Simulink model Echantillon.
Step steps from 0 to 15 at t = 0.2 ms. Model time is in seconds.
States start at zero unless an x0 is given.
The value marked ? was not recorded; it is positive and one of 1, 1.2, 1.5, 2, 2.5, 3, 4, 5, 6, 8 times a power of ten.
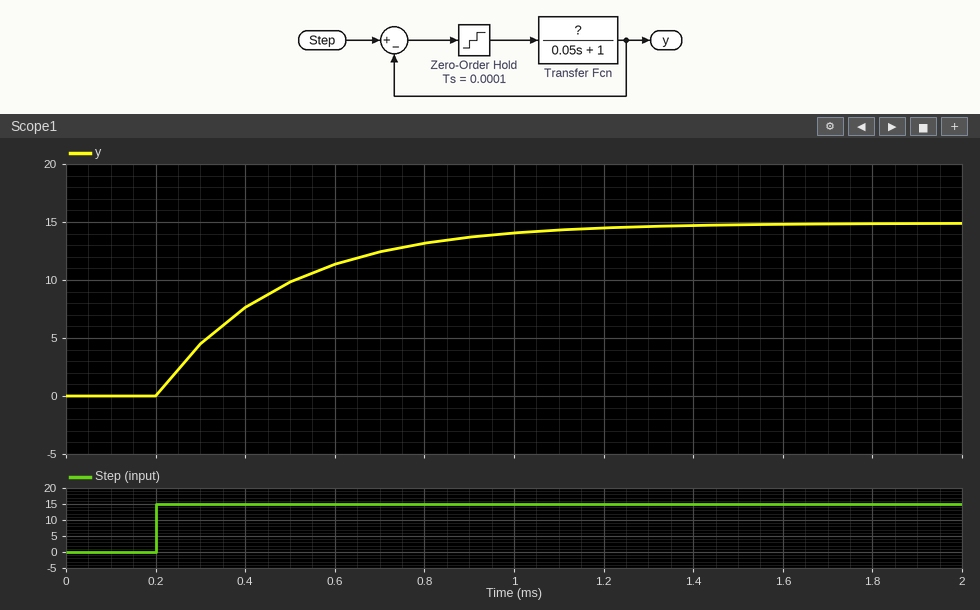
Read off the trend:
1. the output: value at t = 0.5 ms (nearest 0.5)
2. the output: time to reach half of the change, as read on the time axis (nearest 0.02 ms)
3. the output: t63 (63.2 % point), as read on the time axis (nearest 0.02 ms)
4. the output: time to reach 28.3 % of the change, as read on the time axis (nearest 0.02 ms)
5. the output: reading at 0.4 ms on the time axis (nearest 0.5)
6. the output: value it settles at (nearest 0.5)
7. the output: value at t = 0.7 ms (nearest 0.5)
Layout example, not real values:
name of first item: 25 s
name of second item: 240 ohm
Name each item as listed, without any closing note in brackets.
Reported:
the output: value at t = 0.5 ms: 10.0
the output: time to reach half of the change, as read on the time axis: 0.40 ms
the output: t63 (63.2 % point), as read on the time axis: 0.48 ms
the output: time to reach 28.3 % of the change, as read on the time axis: 0.30 ms
the output: reading at 0.4 ms on the time axis: 7.5
the output: value it settles at: 15.0
the output: value at t = 0.7 ms: 12.5
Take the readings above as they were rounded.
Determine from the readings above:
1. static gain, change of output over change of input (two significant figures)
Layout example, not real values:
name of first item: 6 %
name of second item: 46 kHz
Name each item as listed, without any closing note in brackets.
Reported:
static gain, change of output over change of input: 1.0
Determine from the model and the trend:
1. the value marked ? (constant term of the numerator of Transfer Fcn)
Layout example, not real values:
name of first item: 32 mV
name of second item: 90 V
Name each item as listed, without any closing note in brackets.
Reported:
the value marked ?: 150
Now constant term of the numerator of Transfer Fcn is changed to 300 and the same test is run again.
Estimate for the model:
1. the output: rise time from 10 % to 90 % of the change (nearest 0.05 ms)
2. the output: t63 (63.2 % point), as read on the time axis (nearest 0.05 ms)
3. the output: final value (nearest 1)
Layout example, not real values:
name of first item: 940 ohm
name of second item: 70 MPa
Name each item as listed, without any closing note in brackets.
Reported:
the output: rise time from 10 % to 90 % of the change: 0.25 ms
the output: t63 (63.2 % point), as read on the time axis: 0.30 ms
the output: final value: 15
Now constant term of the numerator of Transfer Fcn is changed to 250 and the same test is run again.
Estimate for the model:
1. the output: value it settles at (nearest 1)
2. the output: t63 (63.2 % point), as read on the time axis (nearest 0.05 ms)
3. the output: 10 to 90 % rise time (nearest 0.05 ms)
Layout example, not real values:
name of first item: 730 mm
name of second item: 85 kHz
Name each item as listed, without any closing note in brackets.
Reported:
the output: value it settles at: 15
the output: t63 (63.2 % point), as read on the time axis: 0.35 ms
the output: 10 to 90 % rise time: 0.30 ms
